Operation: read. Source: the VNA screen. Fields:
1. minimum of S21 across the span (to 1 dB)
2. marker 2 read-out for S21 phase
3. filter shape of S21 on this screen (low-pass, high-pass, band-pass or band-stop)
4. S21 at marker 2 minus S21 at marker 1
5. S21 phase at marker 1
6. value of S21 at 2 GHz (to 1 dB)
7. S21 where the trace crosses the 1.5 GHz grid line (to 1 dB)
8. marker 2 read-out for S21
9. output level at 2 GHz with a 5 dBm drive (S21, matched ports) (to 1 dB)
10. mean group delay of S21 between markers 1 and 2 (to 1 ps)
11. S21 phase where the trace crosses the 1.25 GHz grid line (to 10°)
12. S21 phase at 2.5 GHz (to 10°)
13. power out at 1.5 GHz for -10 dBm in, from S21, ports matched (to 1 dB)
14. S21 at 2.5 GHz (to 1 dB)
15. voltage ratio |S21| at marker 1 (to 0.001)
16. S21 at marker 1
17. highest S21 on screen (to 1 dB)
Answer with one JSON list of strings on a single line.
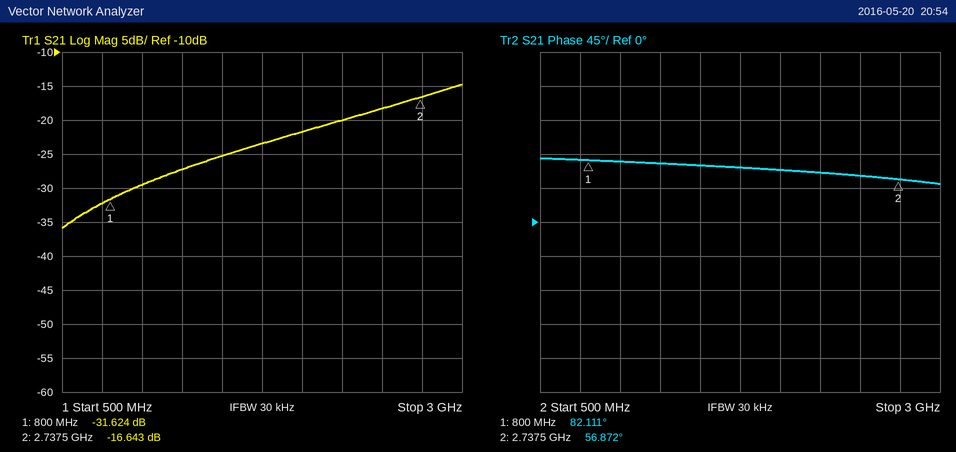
["-36 dB", "56.872°", "high-pass", "14.981 dB", "82.111°", "-22 dB", "-25 dB", "-16.643 dB", "-17 dBm", "36 ps", "80°", "60°", "-35 dBm", "-18 dB", "0.026", "-31.624 dB", "-15 dB"]
